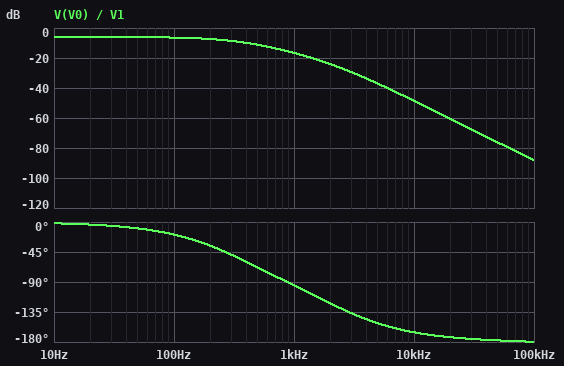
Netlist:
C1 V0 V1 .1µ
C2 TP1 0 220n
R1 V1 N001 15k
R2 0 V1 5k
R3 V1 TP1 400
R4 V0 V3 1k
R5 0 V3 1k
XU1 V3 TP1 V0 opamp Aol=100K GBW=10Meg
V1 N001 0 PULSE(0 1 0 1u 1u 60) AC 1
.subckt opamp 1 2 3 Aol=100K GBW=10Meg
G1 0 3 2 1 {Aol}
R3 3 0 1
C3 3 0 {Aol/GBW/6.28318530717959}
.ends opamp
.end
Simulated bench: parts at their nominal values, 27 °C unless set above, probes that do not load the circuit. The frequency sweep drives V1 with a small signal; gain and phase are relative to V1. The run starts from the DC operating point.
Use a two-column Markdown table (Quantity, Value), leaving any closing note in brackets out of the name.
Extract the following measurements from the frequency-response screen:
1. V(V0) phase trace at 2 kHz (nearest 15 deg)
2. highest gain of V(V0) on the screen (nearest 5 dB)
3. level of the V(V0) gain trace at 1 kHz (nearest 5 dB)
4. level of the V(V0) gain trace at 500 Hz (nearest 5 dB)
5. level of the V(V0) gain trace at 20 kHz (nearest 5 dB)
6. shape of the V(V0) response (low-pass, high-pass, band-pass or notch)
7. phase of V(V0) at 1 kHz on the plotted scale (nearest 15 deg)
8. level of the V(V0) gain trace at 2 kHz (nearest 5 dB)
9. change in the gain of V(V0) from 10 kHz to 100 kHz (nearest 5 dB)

| Quantity | Value |
|---|---|
| V(V0) phase trace at 2 kHz | -120 deg |
| highest gain of V(V0) on the screen | -5 dB |
| level of the V(V0) gain trace at 1 kHz | -15 dB |
| level of the V(V0) gain trace at 500 Hz | -10 dB |
| level of the V(V0) gain trace at 20 kHz | -60 dB |
| shape of the V(V0) response | low-pass |
| phase of V(V0) at 1 kHz on the plotted scale | -90 deg |
| level of the V(V0) gain trace at 2 kHz | -25 dB |
| change in the gain of V(V0) from 10 kHz to 100 kHz | -40 dB |
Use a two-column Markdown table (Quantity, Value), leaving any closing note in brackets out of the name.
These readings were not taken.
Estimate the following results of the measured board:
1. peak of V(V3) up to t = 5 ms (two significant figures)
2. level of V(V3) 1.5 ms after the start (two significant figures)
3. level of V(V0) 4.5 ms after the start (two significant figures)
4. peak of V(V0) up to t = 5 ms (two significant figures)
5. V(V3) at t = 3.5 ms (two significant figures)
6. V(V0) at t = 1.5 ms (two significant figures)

| Quantity | Value |
|---|---|
| peak of V(V3) up to t = 5 ms | 250 mV |
| level of V(V3) 1.5 ms after the start | 240 mV |
| level of V(V0) 4.5 ms after the start | 500 mV |
| peak of V(V0) up to t = 5 ms | 500 mV |
| V(V3) at t = 3.5 ms | 250 mV |
| V(V0) at t = 1.5 ms | 480 mV |
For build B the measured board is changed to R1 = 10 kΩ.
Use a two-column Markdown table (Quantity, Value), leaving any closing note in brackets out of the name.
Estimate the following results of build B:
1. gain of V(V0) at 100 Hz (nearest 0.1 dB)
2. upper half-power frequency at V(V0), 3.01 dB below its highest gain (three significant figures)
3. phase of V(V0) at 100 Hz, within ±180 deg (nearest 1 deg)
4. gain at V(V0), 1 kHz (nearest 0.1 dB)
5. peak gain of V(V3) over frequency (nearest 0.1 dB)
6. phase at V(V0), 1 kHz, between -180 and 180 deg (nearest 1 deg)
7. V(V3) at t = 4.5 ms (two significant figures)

| Quantity | Value |
|---|---|
| gain of V(V0) at 100 Hz | -3.8 dB |
| upper half-power frequency at V(V0), 3.01 dB below its highest gain | 371 Hz |
| phase of V(V0) at 100 Hz, within ±180 deg | -17 deg |
| gain at V(V0), 1 kHz | -13.3 dB |
| peak gain of V(V3) over frequency | -9.5 dB |
| phase at V(V0), 1 kHz, between -180 and 180 deg | -93 deg |
| V(V3) at t = 4.5 ms | 330 mV |
